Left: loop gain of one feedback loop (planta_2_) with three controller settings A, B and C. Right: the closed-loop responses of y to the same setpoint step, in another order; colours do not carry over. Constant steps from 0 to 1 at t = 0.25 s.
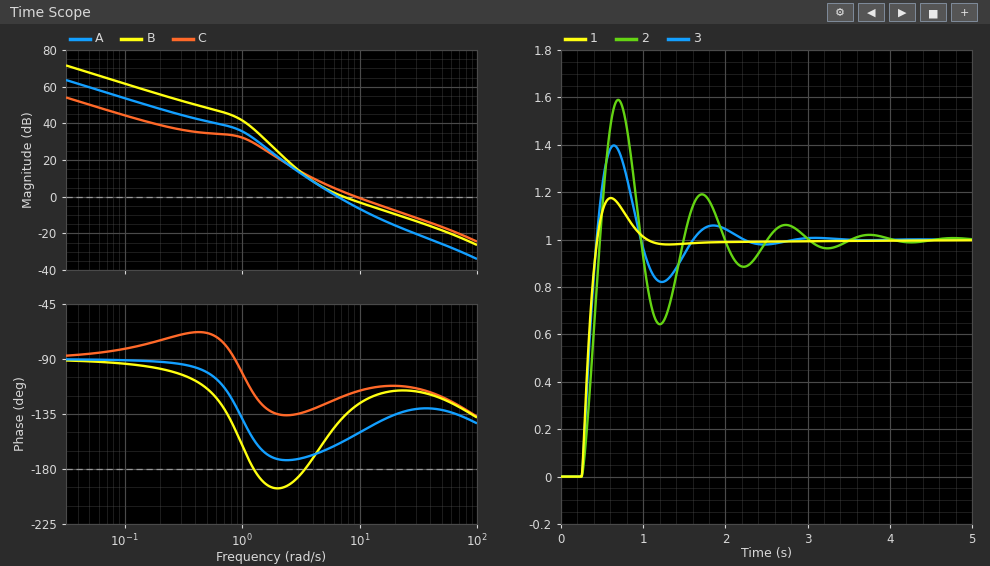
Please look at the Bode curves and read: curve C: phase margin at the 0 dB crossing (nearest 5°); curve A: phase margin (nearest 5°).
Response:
65°
20°
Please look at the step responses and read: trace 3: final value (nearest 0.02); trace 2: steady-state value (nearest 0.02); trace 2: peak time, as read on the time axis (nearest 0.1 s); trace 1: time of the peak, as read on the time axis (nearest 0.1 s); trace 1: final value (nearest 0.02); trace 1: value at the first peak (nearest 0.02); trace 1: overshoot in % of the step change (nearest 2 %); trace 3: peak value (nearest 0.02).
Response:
1.00
1.00
0.7 s
0.6 s
1.00
1.18
18 %
1.40
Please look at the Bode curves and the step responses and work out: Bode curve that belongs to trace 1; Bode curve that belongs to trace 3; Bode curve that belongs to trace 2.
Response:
C
B
A
